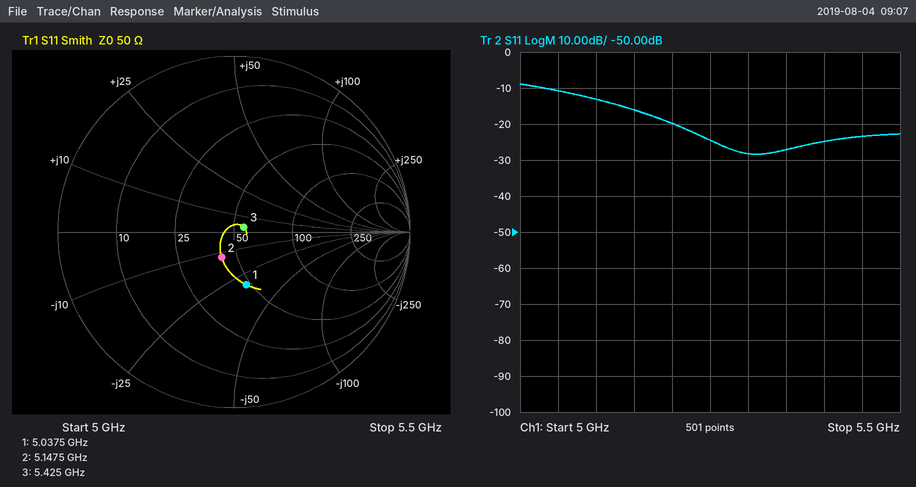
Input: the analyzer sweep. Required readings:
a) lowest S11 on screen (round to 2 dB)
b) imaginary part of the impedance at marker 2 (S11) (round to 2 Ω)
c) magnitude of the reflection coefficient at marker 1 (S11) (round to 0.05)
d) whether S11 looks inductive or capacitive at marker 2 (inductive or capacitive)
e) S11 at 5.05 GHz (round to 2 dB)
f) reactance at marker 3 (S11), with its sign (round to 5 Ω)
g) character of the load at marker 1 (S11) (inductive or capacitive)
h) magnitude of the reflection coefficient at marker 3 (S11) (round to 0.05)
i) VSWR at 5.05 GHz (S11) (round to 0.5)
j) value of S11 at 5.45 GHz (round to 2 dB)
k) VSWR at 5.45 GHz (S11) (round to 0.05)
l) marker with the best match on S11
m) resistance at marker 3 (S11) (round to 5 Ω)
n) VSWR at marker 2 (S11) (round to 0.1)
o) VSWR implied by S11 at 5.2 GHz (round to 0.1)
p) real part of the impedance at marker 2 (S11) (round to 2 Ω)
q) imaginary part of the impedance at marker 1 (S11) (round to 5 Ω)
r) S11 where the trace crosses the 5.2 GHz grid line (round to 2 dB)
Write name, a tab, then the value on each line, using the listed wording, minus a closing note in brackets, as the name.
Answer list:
lowest S11 on screen	-28 dB
imaginary part of the impedance at marker 2 (S11)	-12 Ω
magnitude of the reflection coefficient at marker 1 (S11)	0.30
whether S11 looks inductive or capacitive at marker 2	capacitive
S11 at 5.05 GHz	-10 dB
reactance at marker 3 (S11), with its sign	+5 Ω
character of the load at marker 1 (S11)	capacitive
magnitude of the reflection coefficient at marker 3 (S11)	0.05
VSWR at 5.05 GHz (S11)	2.0
value of S11 at 5.45 GHz	-24 dB
VSWR at 5.45 GHz (S11)	1.15
marker with the best match on S11	marker 3
resistance at marker 3 (S11)	55 Ω
VSWR at marker 2 (S11)	1.4
VSWR implied by S11 at 5.2 GHz	1.2
real part of the impedance at marker 2 (S11)	42 Ω
imaginary part of the impedance at marker 1 (S11)	-30 Ω
S11 where the trace crosses the 5.2 GHz grid line	-20 dB
